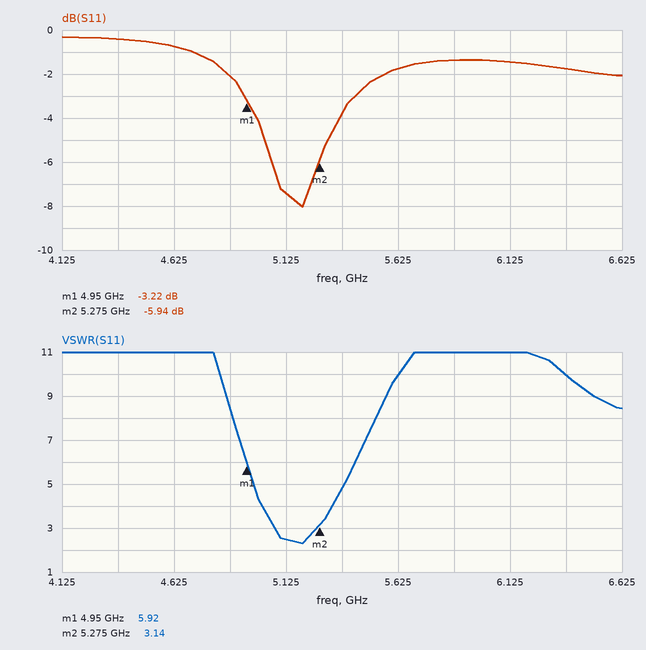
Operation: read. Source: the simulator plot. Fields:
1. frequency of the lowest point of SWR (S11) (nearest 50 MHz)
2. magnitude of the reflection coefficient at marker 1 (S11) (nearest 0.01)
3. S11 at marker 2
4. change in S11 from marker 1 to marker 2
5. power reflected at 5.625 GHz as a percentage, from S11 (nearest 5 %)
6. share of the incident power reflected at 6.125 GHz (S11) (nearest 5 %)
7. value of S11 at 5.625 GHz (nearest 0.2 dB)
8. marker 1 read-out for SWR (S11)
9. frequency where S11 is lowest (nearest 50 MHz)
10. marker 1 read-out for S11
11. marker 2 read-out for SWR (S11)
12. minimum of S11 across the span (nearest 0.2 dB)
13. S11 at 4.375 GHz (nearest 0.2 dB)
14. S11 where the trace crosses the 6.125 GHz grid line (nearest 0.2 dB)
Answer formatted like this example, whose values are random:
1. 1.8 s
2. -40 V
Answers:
1. 5.20 GHz
2. 0.69
3. -5.94 dB
4. -2.72 dB
5. 65 %
6. 70 %
7. -1.8 dB
8. 5.92
9. 5.20 GHz
10. -3.22 dB
11. 3.14
12. -8.0 dB
13. -0.4 dB
14. -1.4 dB
